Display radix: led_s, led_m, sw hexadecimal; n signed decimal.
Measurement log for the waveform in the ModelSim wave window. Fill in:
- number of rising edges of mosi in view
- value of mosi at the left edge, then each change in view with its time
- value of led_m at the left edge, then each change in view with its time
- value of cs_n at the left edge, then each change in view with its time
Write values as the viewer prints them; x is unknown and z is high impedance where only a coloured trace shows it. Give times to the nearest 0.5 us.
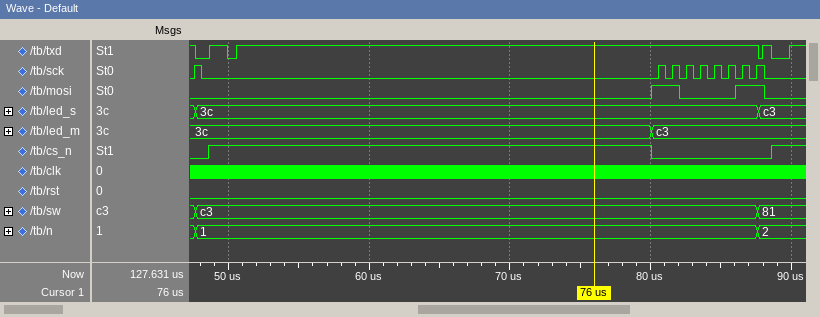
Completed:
2
0, 1 at 80 us, 0 at 82 us, 1 at 86 us, 0 at 88 us
3c, c3 at 80 us
0, 1 at 48.5 us, 0 at 80 us, 1 at 88.5 us
